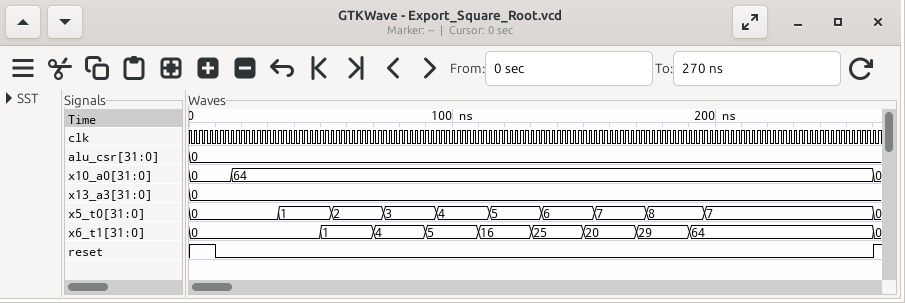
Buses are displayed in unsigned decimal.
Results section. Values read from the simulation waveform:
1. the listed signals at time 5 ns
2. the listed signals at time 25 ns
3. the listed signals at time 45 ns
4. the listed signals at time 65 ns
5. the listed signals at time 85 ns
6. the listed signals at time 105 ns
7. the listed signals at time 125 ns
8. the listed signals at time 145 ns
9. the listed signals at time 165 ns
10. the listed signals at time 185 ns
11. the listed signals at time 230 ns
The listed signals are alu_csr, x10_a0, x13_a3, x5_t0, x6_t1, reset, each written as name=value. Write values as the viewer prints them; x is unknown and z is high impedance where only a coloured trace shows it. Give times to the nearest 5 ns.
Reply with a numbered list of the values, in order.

1. alu_csr=0, x10_a0=0, x13_a3=0, x5_t0=0, x6_t1=0, reset=1
2. alu_csr=0, x10_a0=64, x13_a3=0, x5_t0=0, x6_t1=0, reset=0
3. alu_csr=0, x10_a0=64, x13_a3=0, x5_t0=1, x6_t1=0, reset=0
4. alu_csr=0, x10_a0=64, x13_a3=0, x5_t0=2, x6_t1=1, reset=0
5. alu_csr=0, x10_a0=64, x13_a3=0, x5_t0=3, x6_t1=4, reset=0
6. alu_csr=0, x10_a0=64, x13_a3=0, x5_t0=4, x6_t1=5, reset=0
7. alu_csr=0, x10_a0=64, x13_a3=0, x5_t0=5, x6_t1=16, reset=0
8. alu_csr=0, x10_a0=64, x13_a3=0, x5_t0=6, x6_t1=25, reset=0
9. alu_csr=0, x10_a0=64, x13_a3=0, x5_t0=7, x6_t1=20, reset=0
10. alu_csr=0, x10_a0=64, x13_a3=0, x5_t0=8, x6_t1=29, reset=0
11. alu_csr=0, x10_a0=64, x13_a3=0, x5_t0=7, x6_t1=64, reset=0
